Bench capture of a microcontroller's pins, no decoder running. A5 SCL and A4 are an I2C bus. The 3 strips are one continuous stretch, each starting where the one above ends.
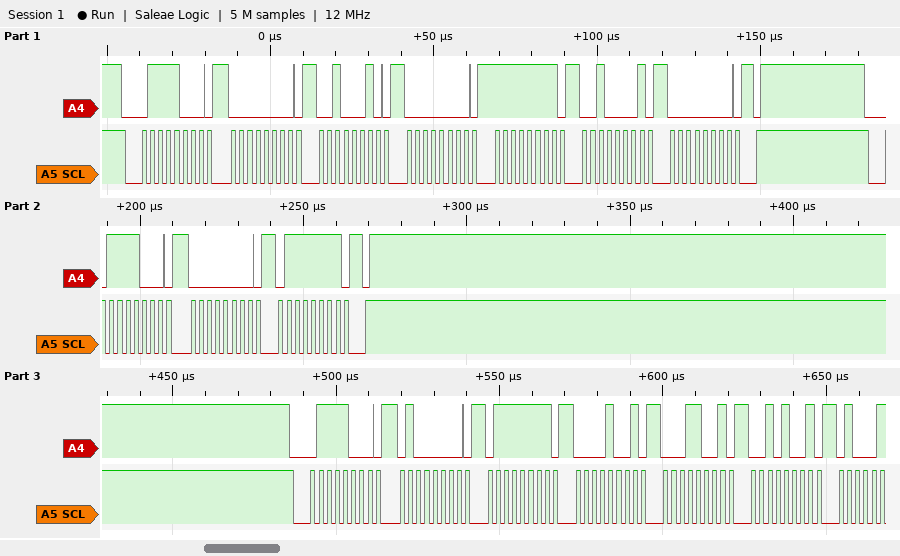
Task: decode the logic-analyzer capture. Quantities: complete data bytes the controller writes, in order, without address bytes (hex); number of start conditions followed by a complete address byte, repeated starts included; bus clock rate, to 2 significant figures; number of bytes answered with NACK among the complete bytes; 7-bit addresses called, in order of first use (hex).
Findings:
00 22 00 FF 21 00 00 7F 40 7F 09 19 29
3
400 kHz
0
0x3C
